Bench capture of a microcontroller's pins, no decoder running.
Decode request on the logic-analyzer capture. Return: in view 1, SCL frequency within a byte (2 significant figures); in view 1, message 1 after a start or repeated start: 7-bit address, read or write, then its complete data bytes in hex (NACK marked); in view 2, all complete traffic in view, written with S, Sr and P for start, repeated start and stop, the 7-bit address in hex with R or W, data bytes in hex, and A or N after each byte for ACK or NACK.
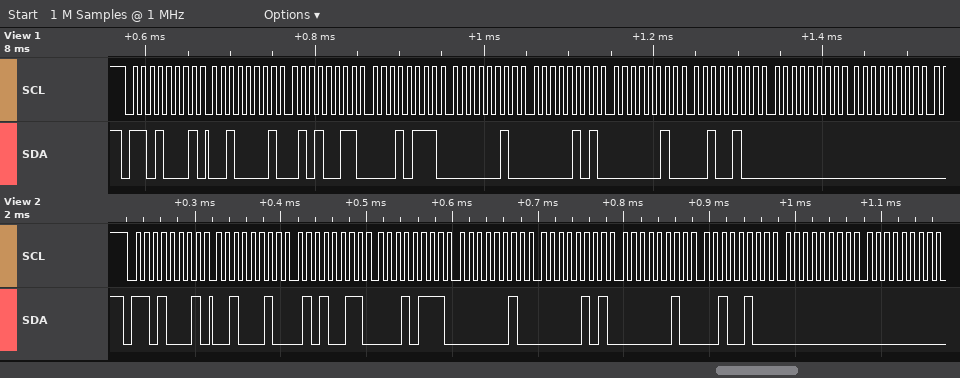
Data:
100 kHz
0x68 read: 21 53 17 02 05 02 24 00 00
S 68R A 22 A 53 A 17 A 02 A 05 A 02 A 24 A 00 A 00 A
